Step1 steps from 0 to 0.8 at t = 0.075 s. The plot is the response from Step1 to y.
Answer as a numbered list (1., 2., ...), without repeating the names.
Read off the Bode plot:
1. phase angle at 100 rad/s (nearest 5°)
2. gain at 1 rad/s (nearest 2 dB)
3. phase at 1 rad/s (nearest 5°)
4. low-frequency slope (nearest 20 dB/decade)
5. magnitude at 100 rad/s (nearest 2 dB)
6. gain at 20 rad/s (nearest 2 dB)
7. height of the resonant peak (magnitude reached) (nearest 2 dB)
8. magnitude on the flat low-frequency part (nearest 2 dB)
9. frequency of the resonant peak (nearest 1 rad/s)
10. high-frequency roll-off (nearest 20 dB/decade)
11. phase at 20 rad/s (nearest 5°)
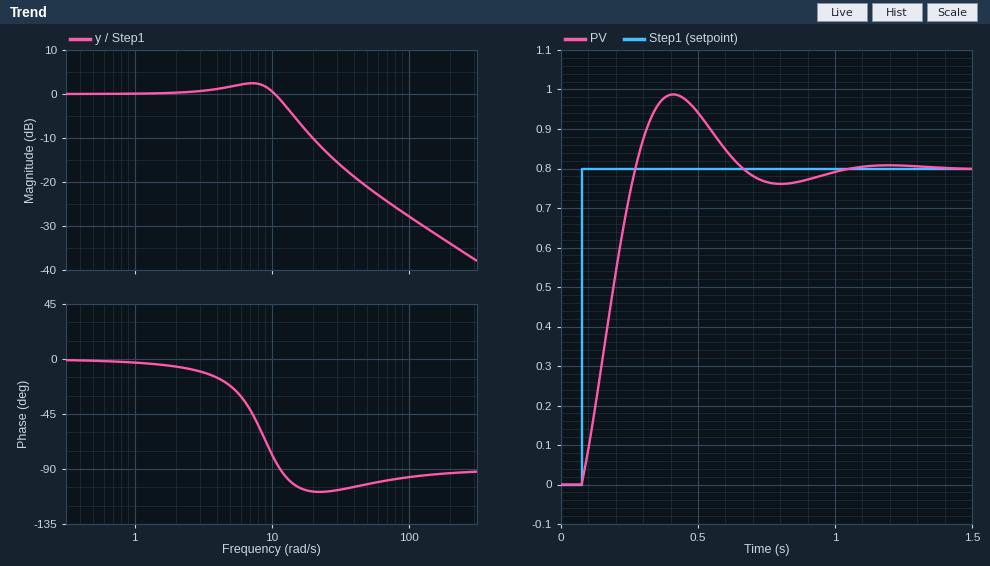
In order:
1. -95°
2. 0 dB
3. -5°
4. 0 dB/decade
5. -28 dB
6. -10 dB
7. 2 dB
8. 0 dB
9. 7 rad/s
10. -20 dB/decade
11. -110°
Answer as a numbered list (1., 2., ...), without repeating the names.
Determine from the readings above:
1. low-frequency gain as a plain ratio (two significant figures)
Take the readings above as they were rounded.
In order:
1. 1.0
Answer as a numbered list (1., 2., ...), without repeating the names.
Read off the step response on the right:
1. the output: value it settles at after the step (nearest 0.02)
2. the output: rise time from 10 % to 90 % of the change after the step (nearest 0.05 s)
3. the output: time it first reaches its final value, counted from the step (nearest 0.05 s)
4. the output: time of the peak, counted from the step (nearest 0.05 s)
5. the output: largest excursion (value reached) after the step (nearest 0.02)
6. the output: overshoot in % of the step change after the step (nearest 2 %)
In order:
1. 0.80
2. 0.15 s
3. 0.20 s
4. 0.35 s
5. 0.98
6. 24 %
